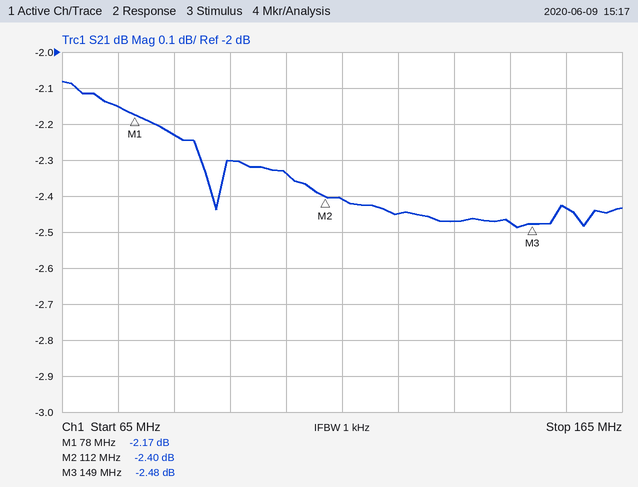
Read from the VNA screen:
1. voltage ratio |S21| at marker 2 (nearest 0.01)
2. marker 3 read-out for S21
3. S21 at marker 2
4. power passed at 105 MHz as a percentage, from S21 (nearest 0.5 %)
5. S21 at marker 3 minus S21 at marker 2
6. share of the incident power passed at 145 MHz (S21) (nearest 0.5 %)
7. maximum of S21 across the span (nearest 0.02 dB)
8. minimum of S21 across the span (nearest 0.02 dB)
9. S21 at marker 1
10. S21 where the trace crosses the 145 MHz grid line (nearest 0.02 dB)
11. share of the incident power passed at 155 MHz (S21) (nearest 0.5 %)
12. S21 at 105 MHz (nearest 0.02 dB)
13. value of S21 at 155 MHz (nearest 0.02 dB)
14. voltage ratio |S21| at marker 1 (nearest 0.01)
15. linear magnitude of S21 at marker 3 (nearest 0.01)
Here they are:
0.76
-2.48 dB
-2.40 dB
58.5 %
-0.08 dB
56.5 %
-2.08 dB
-2.48 dB
-2.17 dB
-2.48 dB
57.0 %
-2.34 dB
-2.44 dB
0.78
0.75
